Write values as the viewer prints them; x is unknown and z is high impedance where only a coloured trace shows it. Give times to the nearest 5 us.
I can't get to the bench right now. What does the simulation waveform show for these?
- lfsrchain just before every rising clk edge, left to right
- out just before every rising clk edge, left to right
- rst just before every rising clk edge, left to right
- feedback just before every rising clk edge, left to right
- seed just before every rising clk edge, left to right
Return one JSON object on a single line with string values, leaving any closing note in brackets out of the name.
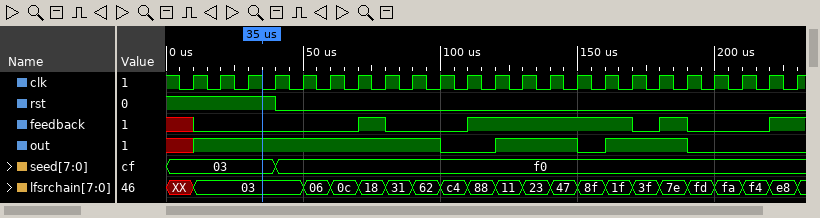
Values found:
{"lfsrchain just before every rising clk edge, left to right": "XX, 03, 03, 03, 03, 06, 0c, 18, 31, 62, c4, 88, 11, 23, 47, 8f, 1f, 3f, 7e, fd, fa, f4, e8", "out just before every rising clk edge, left to right": "x 1 1 1 1 1 1 1 1 1 0 0 1 1 1 0 1 1 1 0 0 0 0", "rst just before every rising clk edge, left to right": "1 1 1 1 0 0 0 0 0 0 0 0 0 0 0 0 0 0 0 0 0 0 0", "feedback just before every rising clk edge, left to right": "x 0 0 0 0 0 0 1 0 0 0 1 1 1 1 1 1 0 1 0 0 0 1", "seed just before every rising clk edge, left to right": "03, 03, 03, 03, f0, f0, f0, f0, f0, f0, f0, f0, f0, f0, f0, f0, f0, f0, f0, f0, f0, f0, f0"}
